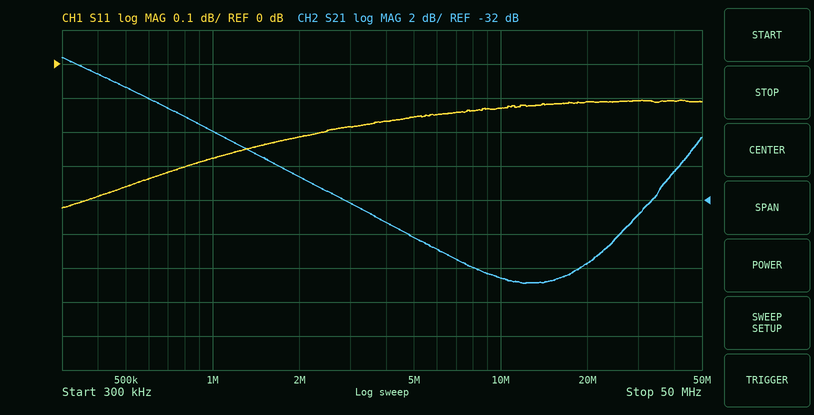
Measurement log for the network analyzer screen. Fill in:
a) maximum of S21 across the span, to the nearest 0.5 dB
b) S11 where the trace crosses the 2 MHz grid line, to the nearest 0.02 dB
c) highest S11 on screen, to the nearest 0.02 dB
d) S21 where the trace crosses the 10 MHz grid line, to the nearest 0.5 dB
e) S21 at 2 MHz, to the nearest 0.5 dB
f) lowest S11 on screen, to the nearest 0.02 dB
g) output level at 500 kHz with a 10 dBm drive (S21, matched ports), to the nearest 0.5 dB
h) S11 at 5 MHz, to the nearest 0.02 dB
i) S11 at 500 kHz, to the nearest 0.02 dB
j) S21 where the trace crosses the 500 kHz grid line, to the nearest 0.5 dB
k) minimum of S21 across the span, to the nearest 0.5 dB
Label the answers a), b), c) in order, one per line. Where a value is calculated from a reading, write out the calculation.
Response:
a) -23.5 dB
b) -0.22 dB
c) -0.10 dB
d) -36.5 dB
e) -30.5 dB
f) -0.42 dB
g) 10 dBm + (-25.5 dB) = -15.5 dBm
h) -0.16 dB
i) -0.36 dB
j) -25.5 dB
k) -37.0 dB
